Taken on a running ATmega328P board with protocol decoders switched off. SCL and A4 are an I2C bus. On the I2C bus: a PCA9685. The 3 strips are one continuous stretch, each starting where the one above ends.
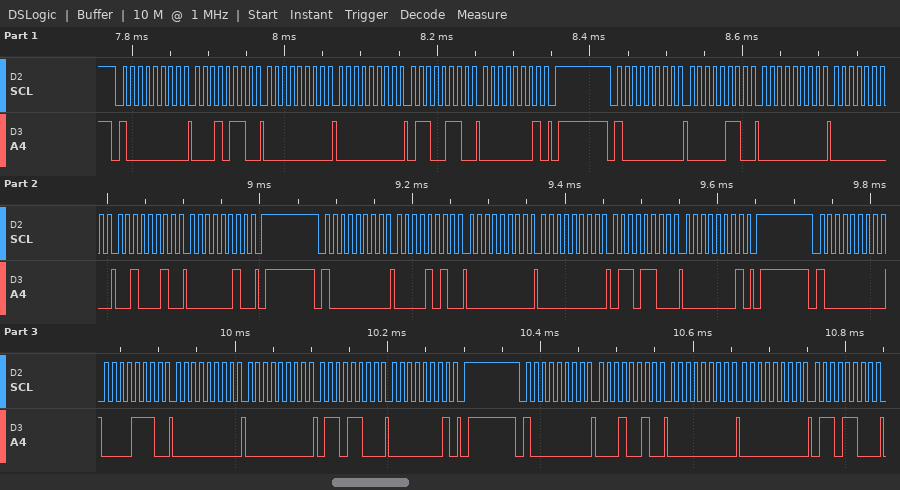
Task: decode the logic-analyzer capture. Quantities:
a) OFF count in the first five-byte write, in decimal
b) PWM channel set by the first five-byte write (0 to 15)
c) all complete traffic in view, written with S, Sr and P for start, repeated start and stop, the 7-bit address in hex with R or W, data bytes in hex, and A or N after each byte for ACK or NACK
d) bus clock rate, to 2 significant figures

358
4
S 40W A 16 A 00 A 00 A 66 A 01 A P S 40W A 06 A 00 A 00 A 22 A 02 A P S 40W A 0A A 00 A 00 A 6C A 01 A P S 40W A 0E A 00 A 00 A 6C A 01 A P S 40W A 12 A 00 A 00 A 6C A
100 kHz
